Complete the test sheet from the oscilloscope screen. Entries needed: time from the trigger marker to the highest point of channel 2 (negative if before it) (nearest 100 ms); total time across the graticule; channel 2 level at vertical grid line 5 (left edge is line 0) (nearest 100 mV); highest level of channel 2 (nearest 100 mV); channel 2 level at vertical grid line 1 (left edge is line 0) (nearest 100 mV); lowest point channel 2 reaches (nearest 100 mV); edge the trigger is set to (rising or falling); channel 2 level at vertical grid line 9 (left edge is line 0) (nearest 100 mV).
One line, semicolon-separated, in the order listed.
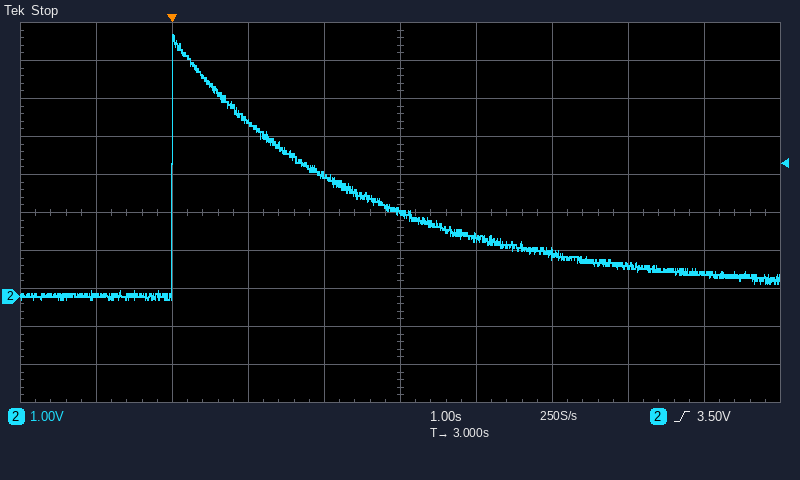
0.0 s; 10 s; 2.2 V; 6.9 V; 0.0 V; -100 mV; rising; 600 mV
